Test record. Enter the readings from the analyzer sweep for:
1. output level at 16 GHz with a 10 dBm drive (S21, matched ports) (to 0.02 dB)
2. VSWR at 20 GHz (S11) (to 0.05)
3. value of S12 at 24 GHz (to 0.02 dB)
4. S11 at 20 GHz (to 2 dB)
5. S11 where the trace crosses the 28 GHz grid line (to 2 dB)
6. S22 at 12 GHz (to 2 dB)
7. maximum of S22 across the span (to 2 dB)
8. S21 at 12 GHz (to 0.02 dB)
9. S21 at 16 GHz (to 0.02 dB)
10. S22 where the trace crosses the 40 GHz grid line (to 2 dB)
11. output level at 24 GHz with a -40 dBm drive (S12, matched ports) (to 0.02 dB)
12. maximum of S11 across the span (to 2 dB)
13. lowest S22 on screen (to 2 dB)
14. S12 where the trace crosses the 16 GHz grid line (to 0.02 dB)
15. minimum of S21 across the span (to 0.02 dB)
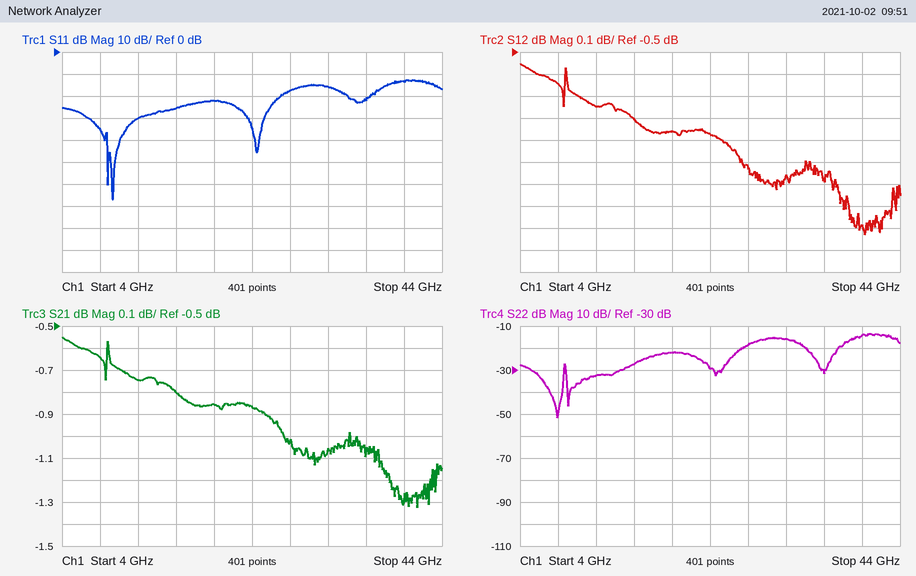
9.20 dBm
1.15
-0.88 dB
-22 dB
-18 dB
-32 dB
-14 dB
-0.74 dB
-0.80 dB
-14 dB
-40.88 dBm
-12 dB
-52 dB
-0.80 dB
-1.32 dB
